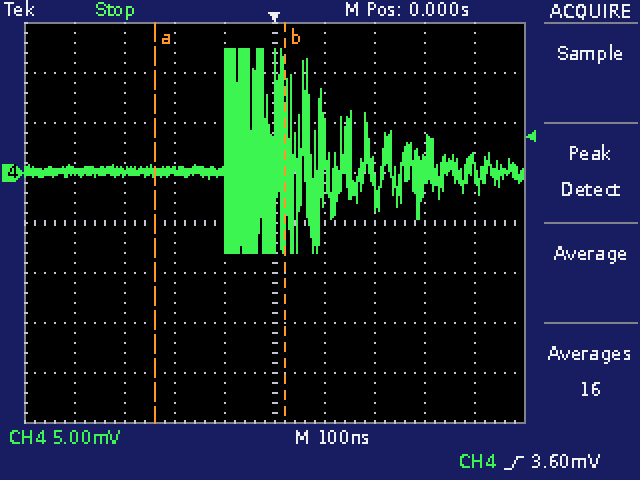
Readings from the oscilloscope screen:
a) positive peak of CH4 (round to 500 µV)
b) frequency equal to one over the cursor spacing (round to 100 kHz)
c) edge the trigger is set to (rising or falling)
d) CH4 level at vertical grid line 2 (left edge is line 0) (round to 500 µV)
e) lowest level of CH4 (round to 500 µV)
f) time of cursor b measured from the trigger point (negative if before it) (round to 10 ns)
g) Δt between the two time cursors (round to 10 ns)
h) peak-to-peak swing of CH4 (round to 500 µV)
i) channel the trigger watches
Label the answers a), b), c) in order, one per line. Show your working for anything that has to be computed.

a) 12.5 mV
b) 1 / 260 ns ≈ 3.8 MHz
c) rising
d) 0.0 mV
e) -8.0 mV
f) +20 ns
g) 260 ns
h) 12.5 mV − (-8.0 mV) = 20.5 mV
i) CH4
